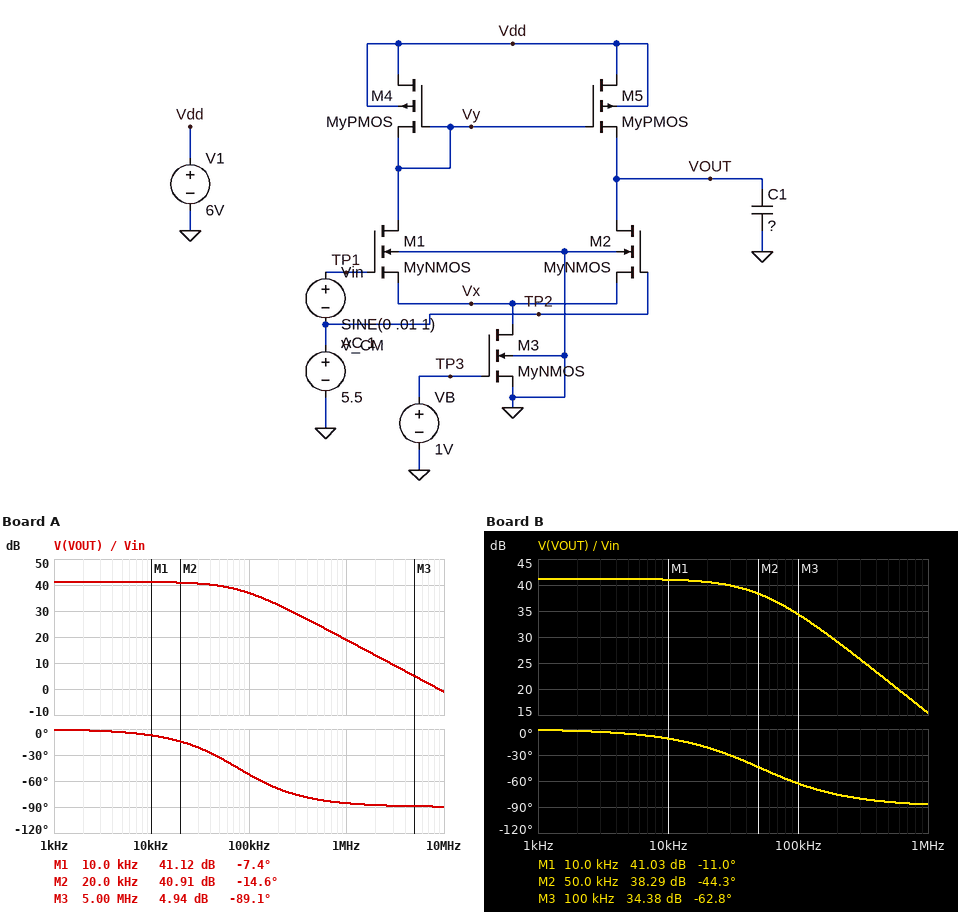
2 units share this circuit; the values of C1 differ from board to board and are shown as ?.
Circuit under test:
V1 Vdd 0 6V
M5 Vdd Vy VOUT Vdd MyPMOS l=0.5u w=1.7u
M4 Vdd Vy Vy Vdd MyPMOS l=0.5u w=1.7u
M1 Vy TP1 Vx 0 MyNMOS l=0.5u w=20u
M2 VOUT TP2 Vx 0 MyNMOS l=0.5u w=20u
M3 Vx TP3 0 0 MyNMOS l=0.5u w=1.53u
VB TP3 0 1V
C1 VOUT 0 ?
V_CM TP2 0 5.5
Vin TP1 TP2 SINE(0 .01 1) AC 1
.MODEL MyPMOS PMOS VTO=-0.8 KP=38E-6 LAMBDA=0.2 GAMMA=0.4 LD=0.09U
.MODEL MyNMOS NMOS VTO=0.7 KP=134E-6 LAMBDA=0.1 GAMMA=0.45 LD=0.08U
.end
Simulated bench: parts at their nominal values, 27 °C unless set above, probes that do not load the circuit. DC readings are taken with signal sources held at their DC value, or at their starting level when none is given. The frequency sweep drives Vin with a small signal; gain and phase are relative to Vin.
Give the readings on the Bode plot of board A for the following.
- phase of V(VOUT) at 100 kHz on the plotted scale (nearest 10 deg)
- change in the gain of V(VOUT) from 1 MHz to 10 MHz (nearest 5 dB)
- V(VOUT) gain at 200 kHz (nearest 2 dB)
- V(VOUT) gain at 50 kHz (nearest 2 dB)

-50 deg
-20 dB
32 dB
40 dB
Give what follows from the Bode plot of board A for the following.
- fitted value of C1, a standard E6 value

10 pF
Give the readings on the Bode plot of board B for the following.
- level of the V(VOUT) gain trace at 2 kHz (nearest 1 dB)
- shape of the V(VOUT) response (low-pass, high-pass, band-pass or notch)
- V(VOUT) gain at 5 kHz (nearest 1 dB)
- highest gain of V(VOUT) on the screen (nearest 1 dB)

41 dB
low-pass
41 dB
41 dB
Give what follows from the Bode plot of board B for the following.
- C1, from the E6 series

15 pF
